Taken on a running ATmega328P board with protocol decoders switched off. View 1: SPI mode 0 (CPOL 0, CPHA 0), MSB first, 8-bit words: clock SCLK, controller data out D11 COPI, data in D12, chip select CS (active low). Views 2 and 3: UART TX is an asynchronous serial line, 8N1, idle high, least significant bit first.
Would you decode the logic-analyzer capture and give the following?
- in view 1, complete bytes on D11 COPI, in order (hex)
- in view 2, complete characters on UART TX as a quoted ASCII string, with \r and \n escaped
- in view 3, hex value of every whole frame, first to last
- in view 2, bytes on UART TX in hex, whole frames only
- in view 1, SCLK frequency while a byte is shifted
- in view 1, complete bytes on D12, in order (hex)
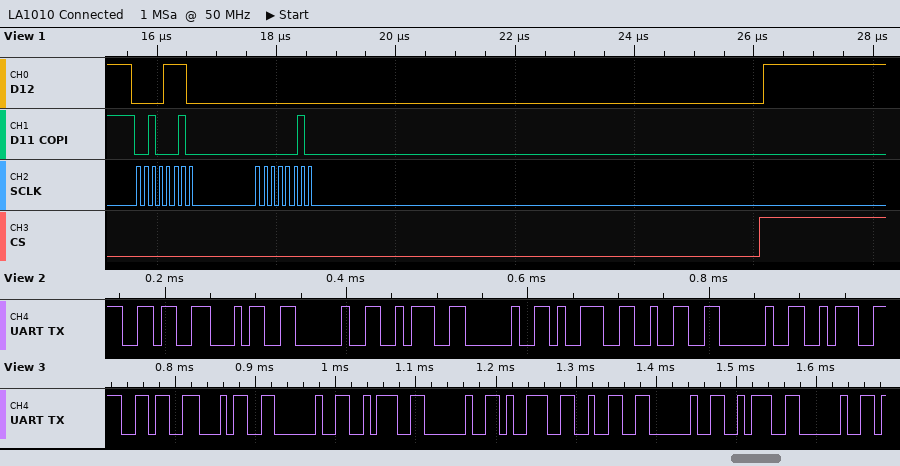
0x22 0x02
"64 : 92 :"
36 34 20 3A 20 39 32 20 3A 20
36 34 20 3A 20 39 32 20 3A
8 MHz
0x0E 0x00
